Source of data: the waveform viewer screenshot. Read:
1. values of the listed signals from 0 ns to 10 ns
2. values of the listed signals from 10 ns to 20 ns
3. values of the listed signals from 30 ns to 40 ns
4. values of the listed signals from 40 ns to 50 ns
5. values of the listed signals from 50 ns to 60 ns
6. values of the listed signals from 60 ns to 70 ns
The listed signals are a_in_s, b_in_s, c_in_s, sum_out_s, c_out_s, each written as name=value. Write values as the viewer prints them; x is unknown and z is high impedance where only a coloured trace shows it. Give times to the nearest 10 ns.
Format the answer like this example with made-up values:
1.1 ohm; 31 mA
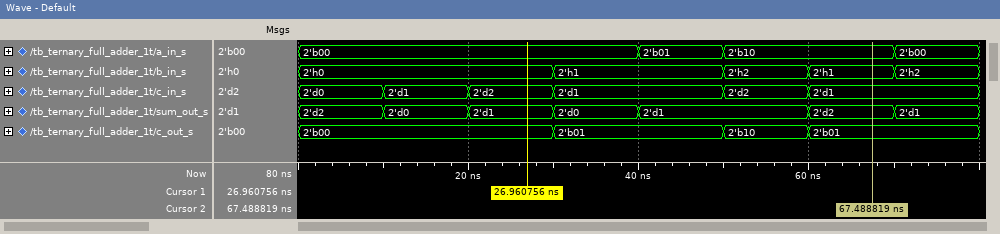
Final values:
a_in_s=2'b00, b_in_s=2'h0, c_in_s=2'd0, sum_out_s=2'd2, c_out_s=2'b00; a_in_s=2'b00, b_in_s=2'h0, c_in_s=2'd1, sum_out_s=2'd0, c_out_s=2'b00; a_in_s=2'b00, b_in_s=2'h1, c_in_s=2'd1, sum_out_s=2'd0, c_out_s=2'b01; a_in_s=2'b01, b_in_s=2'h1, c_in_s=2'd1, sum_out_s=2'd1, c_out_s=2'b01; a_in_s=2'b10, b_in_s=2'h2, c_in_s=2'd2, sum_out_s=2'd1, c_out_s=2'b10; a_in_s=2'b10, b_in_s=2'h1, c_in_s=2'd1, sum_out_s=2'd2, c_out_s=2'b01
